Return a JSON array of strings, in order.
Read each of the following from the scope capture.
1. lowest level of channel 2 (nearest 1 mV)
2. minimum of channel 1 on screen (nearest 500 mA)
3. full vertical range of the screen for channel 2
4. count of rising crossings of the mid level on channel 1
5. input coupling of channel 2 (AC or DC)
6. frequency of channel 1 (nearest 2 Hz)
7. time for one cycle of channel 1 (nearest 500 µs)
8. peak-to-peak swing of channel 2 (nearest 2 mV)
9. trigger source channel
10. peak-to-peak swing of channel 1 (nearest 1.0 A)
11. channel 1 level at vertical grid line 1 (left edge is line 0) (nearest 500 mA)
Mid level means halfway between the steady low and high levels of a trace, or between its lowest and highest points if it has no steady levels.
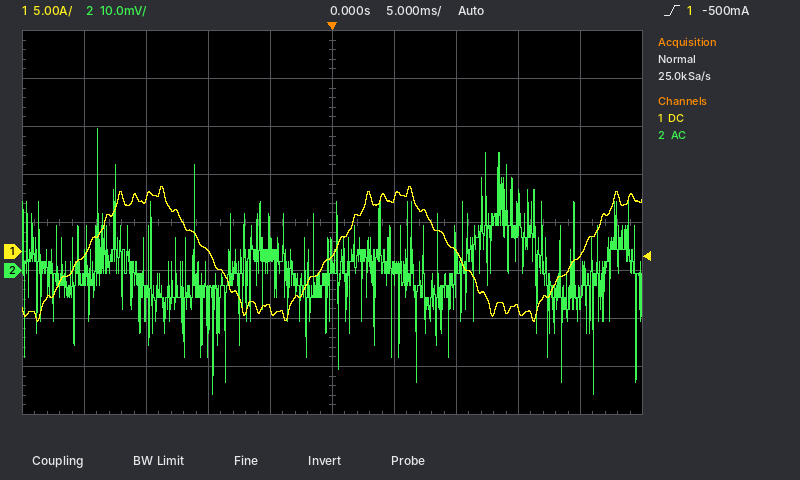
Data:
["-26 mV", "-7.5 A", "80 mV", "3", "AC", "50 Hz", "20.0 ms", "56 mV", "channel 1", "14.0 A", "-500 mA"]
